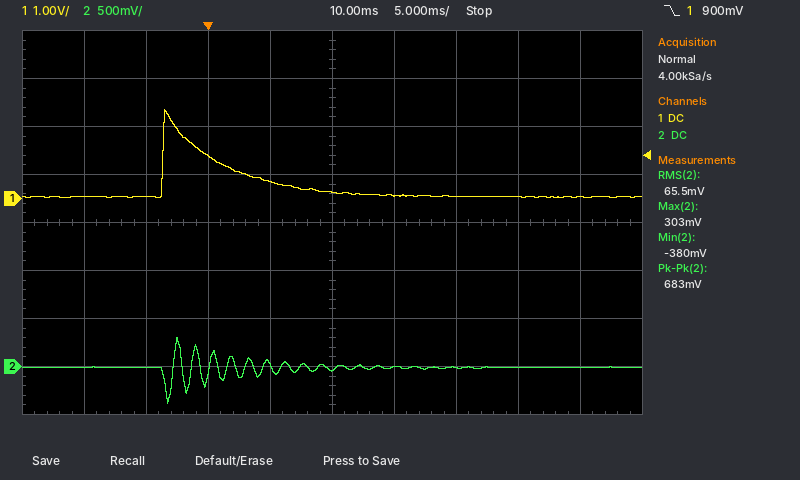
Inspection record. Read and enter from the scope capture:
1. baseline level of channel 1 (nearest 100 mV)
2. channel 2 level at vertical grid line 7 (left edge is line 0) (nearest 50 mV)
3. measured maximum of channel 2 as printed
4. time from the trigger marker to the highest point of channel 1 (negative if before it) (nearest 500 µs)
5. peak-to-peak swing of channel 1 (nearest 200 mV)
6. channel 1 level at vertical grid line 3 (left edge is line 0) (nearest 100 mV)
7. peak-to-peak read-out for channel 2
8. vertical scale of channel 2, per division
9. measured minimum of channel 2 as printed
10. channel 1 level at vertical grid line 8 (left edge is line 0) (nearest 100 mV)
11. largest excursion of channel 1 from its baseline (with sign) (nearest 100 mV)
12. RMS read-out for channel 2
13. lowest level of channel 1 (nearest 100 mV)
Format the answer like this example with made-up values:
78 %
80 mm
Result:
0.0 V
0 mV
303 mV
-3.5 ms
1.8 V
900 mV
683 mV
500 mV
-380 mV
0.0 V
+1.8 V
65.5 mV
0.0 V
